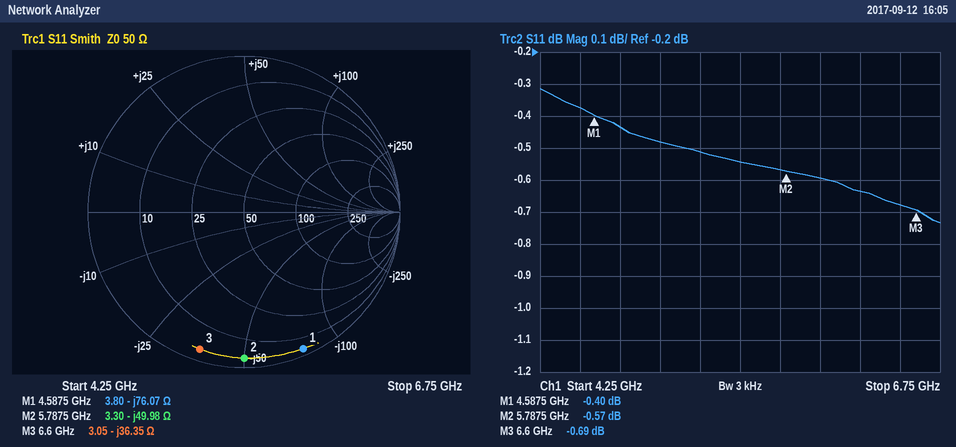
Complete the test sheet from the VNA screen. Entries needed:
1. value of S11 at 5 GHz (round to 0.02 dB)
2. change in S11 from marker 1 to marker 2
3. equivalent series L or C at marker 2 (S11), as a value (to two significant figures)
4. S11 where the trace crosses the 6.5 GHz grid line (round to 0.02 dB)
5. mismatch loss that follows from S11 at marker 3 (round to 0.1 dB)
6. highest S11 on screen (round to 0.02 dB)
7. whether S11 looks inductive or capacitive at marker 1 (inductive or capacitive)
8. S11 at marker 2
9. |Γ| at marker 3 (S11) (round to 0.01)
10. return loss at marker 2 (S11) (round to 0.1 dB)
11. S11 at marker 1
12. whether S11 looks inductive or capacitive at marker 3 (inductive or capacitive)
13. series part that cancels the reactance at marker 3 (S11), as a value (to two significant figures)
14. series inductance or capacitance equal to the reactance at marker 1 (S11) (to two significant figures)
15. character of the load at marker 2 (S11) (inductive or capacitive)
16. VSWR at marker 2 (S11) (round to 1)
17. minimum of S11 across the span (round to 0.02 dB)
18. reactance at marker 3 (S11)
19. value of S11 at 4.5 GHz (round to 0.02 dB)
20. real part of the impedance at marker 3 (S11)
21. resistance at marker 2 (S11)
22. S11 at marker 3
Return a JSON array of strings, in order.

["-0.48 dB", "-0.17 dB", "550 fF", "-0.68 dB", "8.3 dB", "-0.32 dB", "capacitive", "-0.57 dB", "0.92", "0.6 dB", "-0.40 dB", "capacitive", "880 pH", "460 fF", "capacitive", "30", "-0.74 dB", "-36.35 Ω", "-0.38 dB", "3.05 Ω", "3.30 Ω", "-0.69 dB"]
